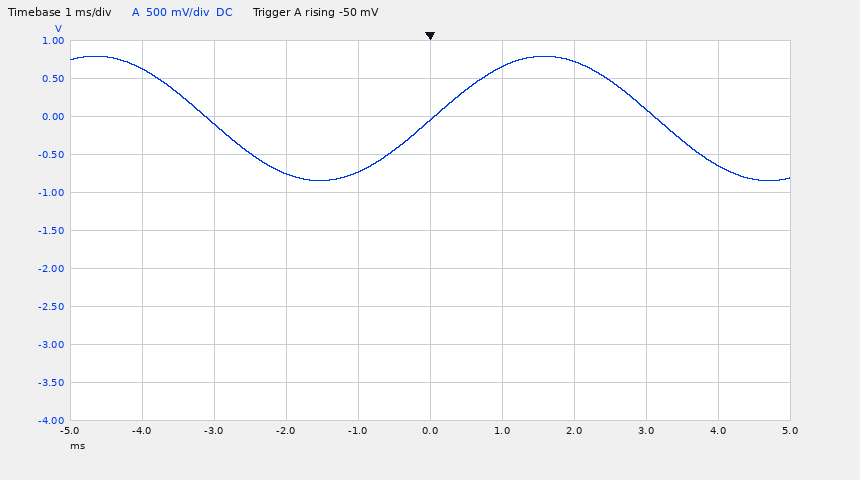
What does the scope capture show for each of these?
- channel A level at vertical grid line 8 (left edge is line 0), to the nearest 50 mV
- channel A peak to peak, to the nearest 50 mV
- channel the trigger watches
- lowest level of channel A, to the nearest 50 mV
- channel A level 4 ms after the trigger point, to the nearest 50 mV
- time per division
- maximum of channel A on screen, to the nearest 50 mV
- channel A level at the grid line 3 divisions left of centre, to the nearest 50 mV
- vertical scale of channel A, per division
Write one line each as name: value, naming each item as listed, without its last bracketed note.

channel A level at vertical grid line 8 (left edge is line 0), to the nearest 50 mV: 100 mV
channel A peak to peak, to the nearest 50 mV: 1.65 V
channel the trigger watches: channel A
lowest level of channel A, to the nearest 50 mV: -850 mV
channel A level 4 ms after the trigger point, to the nearest 50 mV: -650 mV
time per division: 1 ms
maximum of channel A on screen, to the nearest 50 mV: 800 mV
channel A level at the grid line 3 divisions left of centre, to the nearest 50 mV: -100 mV
vertical scale of channel A, per division: 500 mV
